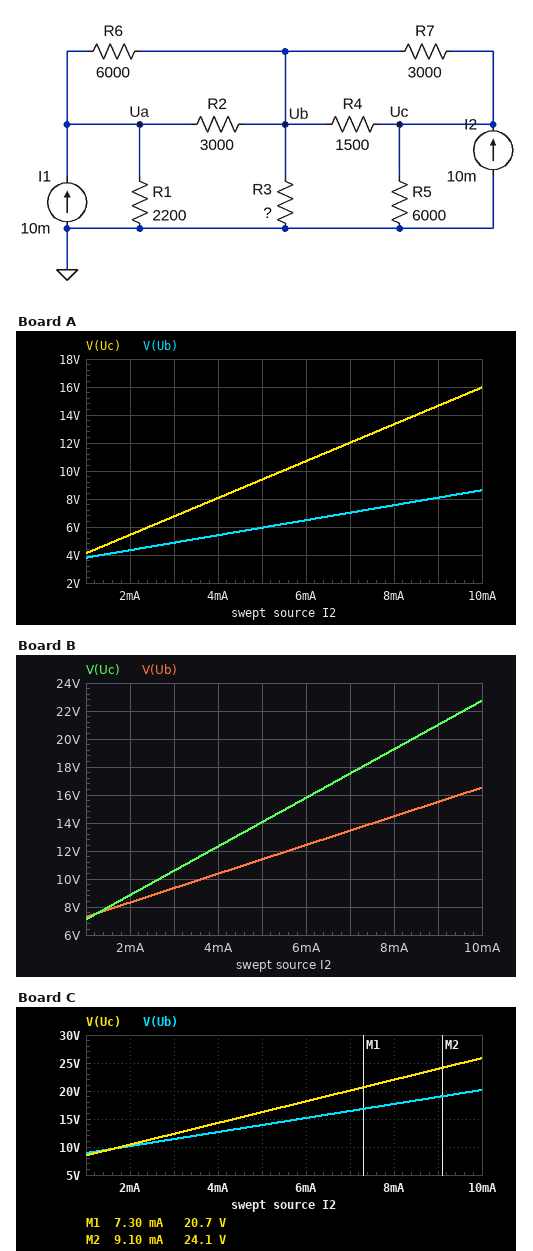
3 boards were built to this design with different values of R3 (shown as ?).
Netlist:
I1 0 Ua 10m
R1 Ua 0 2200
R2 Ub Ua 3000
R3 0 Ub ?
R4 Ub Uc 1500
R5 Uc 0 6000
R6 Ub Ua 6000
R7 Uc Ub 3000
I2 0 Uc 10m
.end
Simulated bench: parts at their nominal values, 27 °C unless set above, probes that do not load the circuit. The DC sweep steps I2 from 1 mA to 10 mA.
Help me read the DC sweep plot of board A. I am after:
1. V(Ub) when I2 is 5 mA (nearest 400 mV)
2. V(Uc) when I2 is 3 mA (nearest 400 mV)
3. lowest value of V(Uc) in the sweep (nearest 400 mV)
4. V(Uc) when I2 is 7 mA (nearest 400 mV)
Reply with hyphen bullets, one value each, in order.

- 6.0 V
- 6.8 V
- 4.0 V
- 12.0 V
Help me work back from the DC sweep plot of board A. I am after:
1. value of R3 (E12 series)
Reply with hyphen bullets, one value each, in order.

- 820 Ω
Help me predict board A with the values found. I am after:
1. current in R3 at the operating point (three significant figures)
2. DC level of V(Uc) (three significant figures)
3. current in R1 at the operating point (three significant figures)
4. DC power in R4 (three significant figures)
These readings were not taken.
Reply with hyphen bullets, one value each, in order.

- 10.5 mA
- 16.0 V
- 6.82 mA
- 35.9 mW
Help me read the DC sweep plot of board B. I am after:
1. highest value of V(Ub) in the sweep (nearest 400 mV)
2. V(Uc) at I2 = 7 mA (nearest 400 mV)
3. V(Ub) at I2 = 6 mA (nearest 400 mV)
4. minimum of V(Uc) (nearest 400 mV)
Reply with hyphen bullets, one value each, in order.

- 16.4 V
- 17.6 V
- 12.4 V
- 7.2 V
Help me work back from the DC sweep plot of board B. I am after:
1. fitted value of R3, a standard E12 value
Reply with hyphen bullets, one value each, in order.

- 2.2 kΩ
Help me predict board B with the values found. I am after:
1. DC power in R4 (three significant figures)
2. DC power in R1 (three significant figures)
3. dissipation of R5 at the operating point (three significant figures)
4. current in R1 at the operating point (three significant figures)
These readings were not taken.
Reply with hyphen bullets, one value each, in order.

- 25.7 mW
- 166 mW
- 86.2 mW
- 8.70 mA
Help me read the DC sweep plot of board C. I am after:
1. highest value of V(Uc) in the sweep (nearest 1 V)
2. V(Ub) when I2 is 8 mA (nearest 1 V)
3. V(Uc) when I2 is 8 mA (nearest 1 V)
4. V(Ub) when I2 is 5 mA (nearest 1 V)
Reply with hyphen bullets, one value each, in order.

- 26 V
- 18 V
- 22 V
- 14 V
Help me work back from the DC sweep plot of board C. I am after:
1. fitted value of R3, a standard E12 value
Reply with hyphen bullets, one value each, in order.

- 3.3 kΩ
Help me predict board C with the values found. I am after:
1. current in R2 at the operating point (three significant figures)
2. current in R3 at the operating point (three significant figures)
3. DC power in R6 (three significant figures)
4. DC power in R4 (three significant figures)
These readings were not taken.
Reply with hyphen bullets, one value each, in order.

- 287 µA
- 6.12 mA
- 124 µW
- 21.6 mW
